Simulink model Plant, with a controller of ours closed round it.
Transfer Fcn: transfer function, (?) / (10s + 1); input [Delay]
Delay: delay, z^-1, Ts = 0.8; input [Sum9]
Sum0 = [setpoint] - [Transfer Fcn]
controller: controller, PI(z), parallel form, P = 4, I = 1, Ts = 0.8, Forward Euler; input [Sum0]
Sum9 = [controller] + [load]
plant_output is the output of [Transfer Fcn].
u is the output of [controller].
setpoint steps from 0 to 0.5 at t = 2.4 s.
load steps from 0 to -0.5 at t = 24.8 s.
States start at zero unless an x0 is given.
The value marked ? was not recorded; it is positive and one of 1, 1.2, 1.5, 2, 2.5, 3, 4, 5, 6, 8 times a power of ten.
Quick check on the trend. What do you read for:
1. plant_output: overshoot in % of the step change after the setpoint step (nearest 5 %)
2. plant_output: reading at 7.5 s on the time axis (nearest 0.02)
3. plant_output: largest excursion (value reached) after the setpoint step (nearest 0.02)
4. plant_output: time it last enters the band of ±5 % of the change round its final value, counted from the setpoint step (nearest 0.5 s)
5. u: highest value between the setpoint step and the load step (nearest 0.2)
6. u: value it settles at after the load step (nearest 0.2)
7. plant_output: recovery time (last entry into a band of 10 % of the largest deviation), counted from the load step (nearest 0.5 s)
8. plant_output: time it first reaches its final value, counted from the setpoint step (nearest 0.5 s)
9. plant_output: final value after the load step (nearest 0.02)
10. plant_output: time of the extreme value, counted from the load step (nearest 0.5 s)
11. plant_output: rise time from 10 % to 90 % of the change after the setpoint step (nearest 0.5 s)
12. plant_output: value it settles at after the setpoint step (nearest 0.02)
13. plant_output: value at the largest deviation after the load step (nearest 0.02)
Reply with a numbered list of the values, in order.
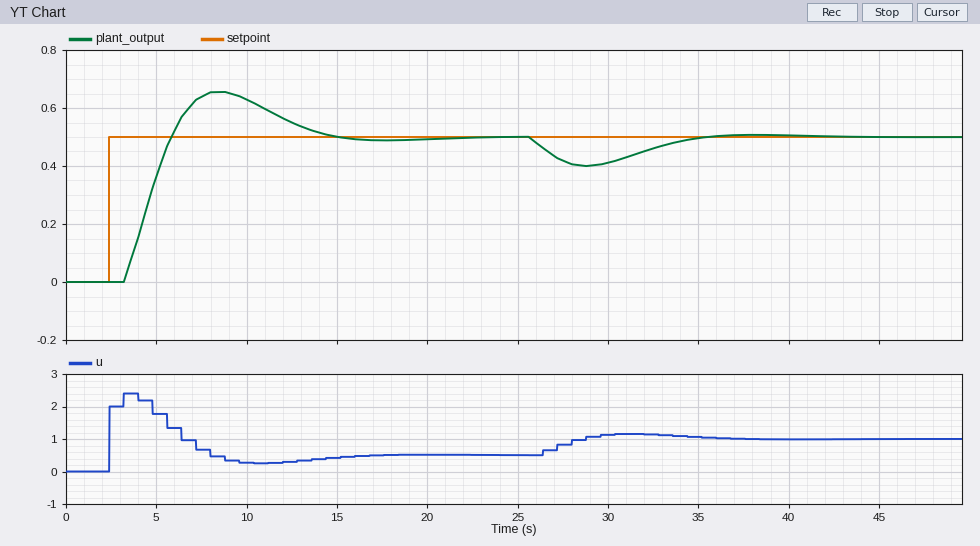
1. 30 %
2. 0.64
3. 0.66
4. 11.0 s
5. 2.4
6. 1.0
7. 9.5 s
8. 3.5 s
9. 0.50
10. 4.0 s
11. 2.0 s
12. 0.50
13. 0.40
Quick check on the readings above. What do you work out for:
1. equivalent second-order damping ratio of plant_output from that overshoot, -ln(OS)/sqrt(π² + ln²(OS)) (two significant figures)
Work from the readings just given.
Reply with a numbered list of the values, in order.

1. 0.36
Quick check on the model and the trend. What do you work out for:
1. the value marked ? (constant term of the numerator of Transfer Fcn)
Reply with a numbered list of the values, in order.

1. 1
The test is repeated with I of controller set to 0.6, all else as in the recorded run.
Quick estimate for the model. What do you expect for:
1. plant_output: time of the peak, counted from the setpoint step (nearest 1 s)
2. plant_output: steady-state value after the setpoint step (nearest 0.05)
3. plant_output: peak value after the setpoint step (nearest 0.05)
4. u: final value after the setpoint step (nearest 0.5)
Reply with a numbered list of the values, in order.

1. 6 s
2. 0.50
3. 0.55
4. 0.5
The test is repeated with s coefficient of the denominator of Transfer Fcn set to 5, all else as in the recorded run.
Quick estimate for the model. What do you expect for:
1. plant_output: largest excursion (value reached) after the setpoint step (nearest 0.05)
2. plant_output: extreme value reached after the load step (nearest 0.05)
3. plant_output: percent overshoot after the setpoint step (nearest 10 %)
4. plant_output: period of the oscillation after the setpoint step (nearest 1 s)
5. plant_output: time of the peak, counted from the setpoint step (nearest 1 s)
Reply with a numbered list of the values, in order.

1. 0.75
2. 0.35
3. 50 %
4. 6 s
5. 3 s
